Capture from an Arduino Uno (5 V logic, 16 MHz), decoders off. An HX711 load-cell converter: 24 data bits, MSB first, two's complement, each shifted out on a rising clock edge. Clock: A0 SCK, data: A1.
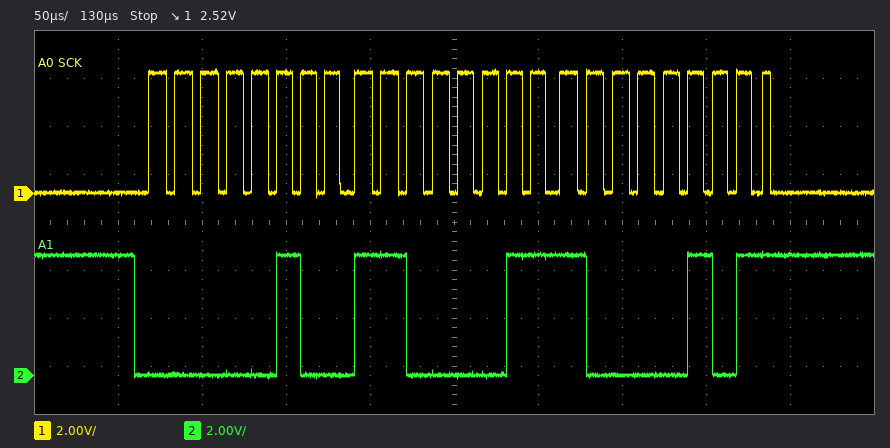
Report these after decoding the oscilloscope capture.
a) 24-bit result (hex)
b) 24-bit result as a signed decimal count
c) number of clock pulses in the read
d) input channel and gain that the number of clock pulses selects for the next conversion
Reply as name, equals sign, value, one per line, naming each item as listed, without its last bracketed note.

24-bit result = 0x04C385
24-bit result as a signed decimal count = 312197
number of clock pulses in the read = 25
input channel and gain that the number of clock pulses selects for the next conversion = channel A, gain 128
